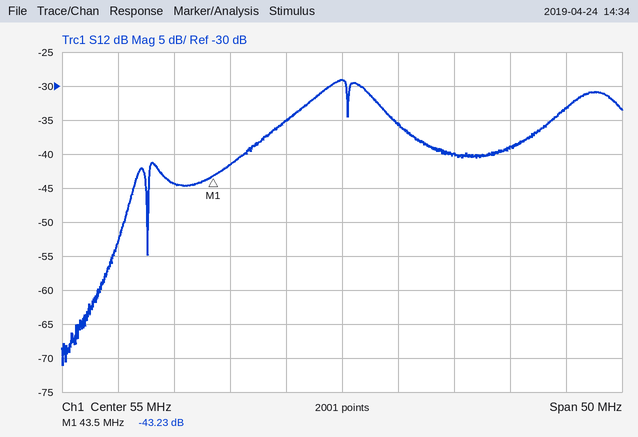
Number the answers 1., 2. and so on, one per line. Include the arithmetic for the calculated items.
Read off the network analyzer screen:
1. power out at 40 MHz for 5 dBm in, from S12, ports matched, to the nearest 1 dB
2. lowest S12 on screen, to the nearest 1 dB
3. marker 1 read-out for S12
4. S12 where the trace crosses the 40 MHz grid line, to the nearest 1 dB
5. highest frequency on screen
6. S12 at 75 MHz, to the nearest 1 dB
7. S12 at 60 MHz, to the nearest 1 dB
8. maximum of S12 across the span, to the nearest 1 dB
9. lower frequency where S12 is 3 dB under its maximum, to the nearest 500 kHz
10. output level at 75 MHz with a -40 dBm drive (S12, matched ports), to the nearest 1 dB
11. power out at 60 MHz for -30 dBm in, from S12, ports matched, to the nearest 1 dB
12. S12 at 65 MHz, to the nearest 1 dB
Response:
1. 5 dBm + (-44 dB) = -39 dBm
2. -71 dB
3. -43.23 dB
4. -44 dB
5. 80 MHz
6. -33 dB
7. -36 dB
8. -29 dB
9. 52.5 MHz
10. -40 dBm + (-33 dB) = -73 dBm
11. -30 dBm + (-36 dB) = -66 dBm
12. -40 dB
